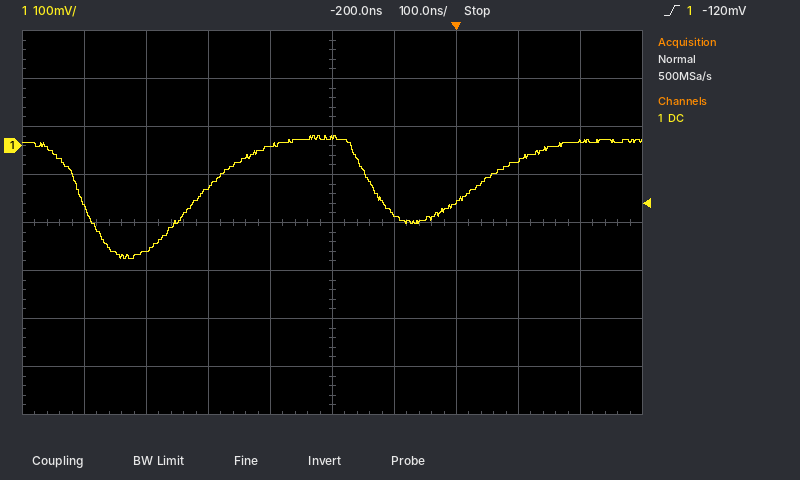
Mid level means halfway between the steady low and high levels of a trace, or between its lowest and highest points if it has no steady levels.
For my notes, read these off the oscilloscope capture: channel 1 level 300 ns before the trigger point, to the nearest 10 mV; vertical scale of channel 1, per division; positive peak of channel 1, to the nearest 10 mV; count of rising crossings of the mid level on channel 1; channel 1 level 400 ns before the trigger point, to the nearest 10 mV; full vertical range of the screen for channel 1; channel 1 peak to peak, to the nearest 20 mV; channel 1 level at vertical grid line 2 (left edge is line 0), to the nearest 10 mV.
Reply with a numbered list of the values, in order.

1. 0 mV
2. 100 mV
3. 20 mV
4. 2
5. -90 mV
6. 800 mV
7. 260 mV
8. -220 mV
